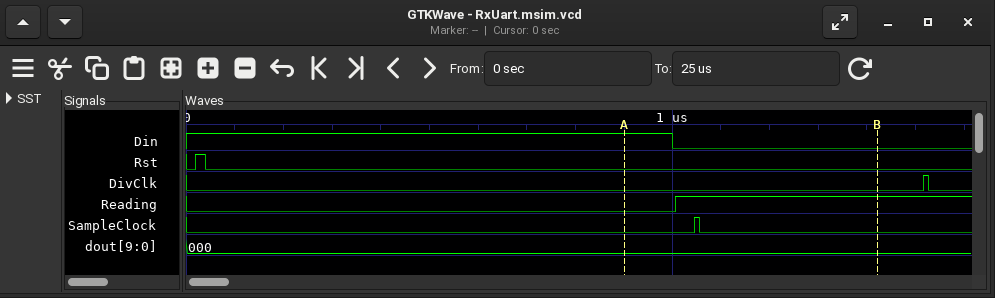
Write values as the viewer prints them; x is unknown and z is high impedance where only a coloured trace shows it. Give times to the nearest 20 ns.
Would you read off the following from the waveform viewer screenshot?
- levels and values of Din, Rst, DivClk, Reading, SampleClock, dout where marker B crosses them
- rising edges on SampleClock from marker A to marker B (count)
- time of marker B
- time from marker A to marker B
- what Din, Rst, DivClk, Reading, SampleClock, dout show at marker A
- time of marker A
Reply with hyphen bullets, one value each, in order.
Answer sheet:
- Din=0, Rst=0, DivClk=0, Reading=1, SampleClock=0, dout=000
- 1
- 1420 ns
- 520 ns
- Din=1, Rst=0, DivClk=0, Reading=0, SampleClock=0, dout=000
- 900 ns
